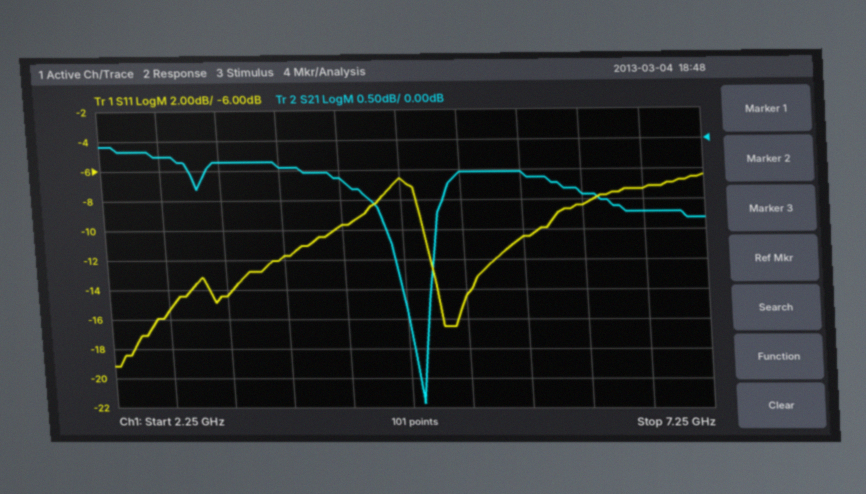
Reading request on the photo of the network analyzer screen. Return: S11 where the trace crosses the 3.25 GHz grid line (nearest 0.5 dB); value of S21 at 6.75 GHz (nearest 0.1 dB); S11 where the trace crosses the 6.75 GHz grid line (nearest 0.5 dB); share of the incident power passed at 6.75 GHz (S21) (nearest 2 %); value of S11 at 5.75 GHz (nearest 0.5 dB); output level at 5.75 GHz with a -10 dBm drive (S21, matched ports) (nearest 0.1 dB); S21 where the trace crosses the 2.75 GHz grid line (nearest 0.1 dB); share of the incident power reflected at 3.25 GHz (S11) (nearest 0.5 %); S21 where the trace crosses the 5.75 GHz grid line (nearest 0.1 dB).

-14.5 dB
-1.2 dB
-7.5 dB
76 %
-10.5 dB
-10.5 dBm
-0.3 dB
3.5 %
-0.5 dB
